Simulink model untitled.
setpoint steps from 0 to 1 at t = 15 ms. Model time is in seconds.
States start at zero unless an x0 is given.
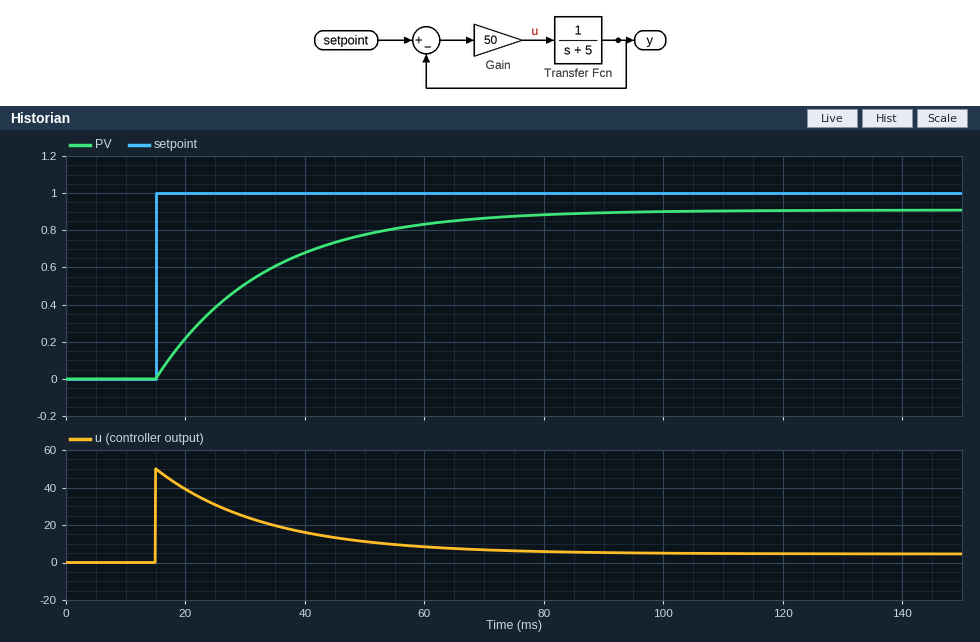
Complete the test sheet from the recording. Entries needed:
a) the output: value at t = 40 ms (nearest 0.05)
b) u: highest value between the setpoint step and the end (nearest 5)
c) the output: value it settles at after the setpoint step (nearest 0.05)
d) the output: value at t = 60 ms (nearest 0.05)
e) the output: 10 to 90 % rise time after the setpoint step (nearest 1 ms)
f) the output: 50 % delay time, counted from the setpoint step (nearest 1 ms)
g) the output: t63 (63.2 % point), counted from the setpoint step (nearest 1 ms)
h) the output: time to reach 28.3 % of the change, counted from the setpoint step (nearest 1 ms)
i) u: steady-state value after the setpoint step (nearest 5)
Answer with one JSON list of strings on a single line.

["0.70", "50", "0.90", "0.85", "40 ms", "13 ms", "18 ms", "6 ms", "5"]
